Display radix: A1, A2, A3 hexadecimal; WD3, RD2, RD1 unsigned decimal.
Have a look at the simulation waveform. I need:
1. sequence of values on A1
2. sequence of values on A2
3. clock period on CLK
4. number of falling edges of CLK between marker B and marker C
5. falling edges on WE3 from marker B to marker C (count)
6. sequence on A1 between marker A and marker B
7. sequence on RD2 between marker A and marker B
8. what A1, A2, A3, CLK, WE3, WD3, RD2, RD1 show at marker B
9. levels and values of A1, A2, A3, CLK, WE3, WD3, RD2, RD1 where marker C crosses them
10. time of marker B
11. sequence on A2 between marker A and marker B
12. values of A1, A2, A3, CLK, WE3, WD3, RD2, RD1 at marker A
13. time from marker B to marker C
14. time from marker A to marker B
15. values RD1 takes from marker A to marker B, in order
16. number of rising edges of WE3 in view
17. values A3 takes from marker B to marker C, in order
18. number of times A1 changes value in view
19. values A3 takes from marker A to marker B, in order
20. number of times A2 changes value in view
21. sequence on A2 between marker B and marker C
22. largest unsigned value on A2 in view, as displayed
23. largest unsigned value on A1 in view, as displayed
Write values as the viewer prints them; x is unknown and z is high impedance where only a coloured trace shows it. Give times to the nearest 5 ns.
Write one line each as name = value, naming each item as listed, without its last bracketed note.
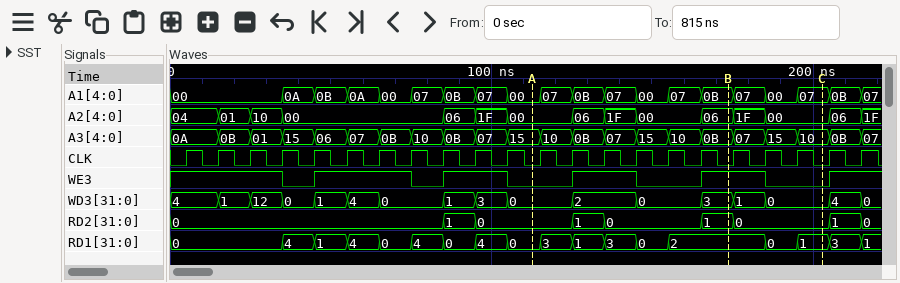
sequence of values on A1 = 00, 0A, 0B, 0A, 00, 07, 0B, 07, 00, 07, 0B, 07, 00, 07, 0B, 07, 00, 07, 0B, 07
sequence of values on A2 = 04, 01, 10, 00, 06, 1F, 00, 06, 1F, 00, 06, 1F, 00, 06, 1F
clock period on CLK = 10 ns
number of falling edges of CLK between marker B and marker C = 3
falling edges on WE3 from marker B to marker C = 1
sequence on A1 between marker A and marker B = 00, 07, 0B, 07, 00, 07, 0B
sequence on RD2 between marker A and marker B = 0, 1, 0, 1
what A1, A2, A3, CLK, WE3, WD3, RD2, RD1 show at marker B = A1=0B, A2=06, A3=0B, CLK=0, WE3=1, WD3=3, RD2=1, RD1=2
levels and values of A1, A2, A3, CLK, WE3, WD3, RD2, RD1 where marker C crosses them = A1=07, A2=00, A3=10, CLK=0, WE3=0, WD3=0, RD2=0, RD1=1
time of marker B = 175 ns
sequence on A2 between marker A and marker B = 00, 06, 1F, 00, 06
values of A1, A2, A3, CLK, WE3, WD3, RD2, RD1 at marker A = A1=00, A2=00, A3=15, CLK=0, WE3=0, WD3=0, RD2=0, RD1=0
time from marker B to marker C = 30 ns
time from marker A to marker B = 60 ns
values RD1 takes from marker A to marker B, in order = 0, 3, 1, 3, 0, 2
number of rising edges of WE3 in view = 5
values A3 takes from marker B to marker C, in order = 0B, 07, 15, 10
number of times A1 changes value in view = 19
values A3 takes from marker A to marker B, in order = 15, 10, 0B, 07, 15, 10, 0B
number of times A2 changes value in view = 14
sequence on A2 between marker B and marker C = 06, 1F, 00
largest unsigned value on A2 in view, as displayed = 1F
largest unsigned value on A1 in view, as displayed = 0B
